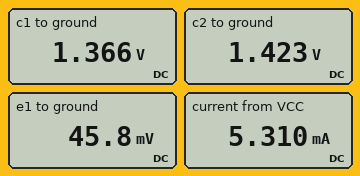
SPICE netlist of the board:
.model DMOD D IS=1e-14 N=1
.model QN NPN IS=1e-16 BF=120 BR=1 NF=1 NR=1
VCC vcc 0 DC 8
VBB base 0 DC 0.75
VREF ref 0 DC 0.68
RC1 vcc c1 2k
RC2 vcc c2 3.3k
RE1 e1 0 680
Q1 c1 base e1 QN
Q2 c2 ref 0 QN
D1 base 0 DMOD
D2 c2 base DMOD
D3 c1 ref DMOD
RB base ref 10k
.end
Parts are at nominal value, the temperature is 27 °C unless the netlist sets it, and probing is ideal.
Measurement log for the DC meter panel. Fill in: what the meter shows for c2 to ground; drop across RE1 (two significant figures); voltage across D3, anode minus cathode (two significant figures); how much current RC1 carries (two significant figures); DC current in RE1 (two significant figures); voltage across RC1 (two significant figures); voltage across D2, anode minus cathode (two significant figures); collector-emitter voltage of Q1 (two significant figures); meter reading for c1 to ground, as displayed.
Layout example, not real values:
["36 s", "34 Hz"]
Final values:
["1.423 V", "46 mV", "690 mV", "3.3 mA", "67 µA", "6.6 V", "670 mV", "1.3 V", "1.366 V"]
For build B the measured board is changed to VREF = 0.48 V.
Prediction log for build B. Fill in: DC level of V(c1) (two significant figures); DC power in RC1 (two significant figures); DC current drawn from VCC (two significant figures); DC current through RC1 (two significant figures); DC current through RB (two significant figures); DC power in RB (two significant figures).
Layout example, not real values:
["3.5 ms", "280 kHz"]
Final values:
["1.2 V", "23 mW", "5.4 mA", "3.4 mA", "27 µA", "7.3 µW"]
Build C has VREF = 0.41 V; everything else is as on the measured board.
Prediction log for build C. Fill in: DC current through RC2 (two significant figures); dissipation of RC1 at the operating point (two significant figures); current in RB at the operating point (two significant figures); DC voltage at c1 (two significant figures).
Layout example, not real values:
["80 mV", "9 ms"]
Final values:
["2.0 mA", "24 mW", "34 µA", "1.1 V"]
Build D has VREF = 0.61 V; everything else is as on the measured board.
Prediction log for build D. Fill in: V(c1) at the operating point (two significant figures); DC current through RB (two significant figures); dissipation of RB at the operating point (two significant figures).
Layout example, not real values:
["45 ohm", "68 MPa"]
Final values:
["1.3 V", "14 µA", "2.0 µW"]
